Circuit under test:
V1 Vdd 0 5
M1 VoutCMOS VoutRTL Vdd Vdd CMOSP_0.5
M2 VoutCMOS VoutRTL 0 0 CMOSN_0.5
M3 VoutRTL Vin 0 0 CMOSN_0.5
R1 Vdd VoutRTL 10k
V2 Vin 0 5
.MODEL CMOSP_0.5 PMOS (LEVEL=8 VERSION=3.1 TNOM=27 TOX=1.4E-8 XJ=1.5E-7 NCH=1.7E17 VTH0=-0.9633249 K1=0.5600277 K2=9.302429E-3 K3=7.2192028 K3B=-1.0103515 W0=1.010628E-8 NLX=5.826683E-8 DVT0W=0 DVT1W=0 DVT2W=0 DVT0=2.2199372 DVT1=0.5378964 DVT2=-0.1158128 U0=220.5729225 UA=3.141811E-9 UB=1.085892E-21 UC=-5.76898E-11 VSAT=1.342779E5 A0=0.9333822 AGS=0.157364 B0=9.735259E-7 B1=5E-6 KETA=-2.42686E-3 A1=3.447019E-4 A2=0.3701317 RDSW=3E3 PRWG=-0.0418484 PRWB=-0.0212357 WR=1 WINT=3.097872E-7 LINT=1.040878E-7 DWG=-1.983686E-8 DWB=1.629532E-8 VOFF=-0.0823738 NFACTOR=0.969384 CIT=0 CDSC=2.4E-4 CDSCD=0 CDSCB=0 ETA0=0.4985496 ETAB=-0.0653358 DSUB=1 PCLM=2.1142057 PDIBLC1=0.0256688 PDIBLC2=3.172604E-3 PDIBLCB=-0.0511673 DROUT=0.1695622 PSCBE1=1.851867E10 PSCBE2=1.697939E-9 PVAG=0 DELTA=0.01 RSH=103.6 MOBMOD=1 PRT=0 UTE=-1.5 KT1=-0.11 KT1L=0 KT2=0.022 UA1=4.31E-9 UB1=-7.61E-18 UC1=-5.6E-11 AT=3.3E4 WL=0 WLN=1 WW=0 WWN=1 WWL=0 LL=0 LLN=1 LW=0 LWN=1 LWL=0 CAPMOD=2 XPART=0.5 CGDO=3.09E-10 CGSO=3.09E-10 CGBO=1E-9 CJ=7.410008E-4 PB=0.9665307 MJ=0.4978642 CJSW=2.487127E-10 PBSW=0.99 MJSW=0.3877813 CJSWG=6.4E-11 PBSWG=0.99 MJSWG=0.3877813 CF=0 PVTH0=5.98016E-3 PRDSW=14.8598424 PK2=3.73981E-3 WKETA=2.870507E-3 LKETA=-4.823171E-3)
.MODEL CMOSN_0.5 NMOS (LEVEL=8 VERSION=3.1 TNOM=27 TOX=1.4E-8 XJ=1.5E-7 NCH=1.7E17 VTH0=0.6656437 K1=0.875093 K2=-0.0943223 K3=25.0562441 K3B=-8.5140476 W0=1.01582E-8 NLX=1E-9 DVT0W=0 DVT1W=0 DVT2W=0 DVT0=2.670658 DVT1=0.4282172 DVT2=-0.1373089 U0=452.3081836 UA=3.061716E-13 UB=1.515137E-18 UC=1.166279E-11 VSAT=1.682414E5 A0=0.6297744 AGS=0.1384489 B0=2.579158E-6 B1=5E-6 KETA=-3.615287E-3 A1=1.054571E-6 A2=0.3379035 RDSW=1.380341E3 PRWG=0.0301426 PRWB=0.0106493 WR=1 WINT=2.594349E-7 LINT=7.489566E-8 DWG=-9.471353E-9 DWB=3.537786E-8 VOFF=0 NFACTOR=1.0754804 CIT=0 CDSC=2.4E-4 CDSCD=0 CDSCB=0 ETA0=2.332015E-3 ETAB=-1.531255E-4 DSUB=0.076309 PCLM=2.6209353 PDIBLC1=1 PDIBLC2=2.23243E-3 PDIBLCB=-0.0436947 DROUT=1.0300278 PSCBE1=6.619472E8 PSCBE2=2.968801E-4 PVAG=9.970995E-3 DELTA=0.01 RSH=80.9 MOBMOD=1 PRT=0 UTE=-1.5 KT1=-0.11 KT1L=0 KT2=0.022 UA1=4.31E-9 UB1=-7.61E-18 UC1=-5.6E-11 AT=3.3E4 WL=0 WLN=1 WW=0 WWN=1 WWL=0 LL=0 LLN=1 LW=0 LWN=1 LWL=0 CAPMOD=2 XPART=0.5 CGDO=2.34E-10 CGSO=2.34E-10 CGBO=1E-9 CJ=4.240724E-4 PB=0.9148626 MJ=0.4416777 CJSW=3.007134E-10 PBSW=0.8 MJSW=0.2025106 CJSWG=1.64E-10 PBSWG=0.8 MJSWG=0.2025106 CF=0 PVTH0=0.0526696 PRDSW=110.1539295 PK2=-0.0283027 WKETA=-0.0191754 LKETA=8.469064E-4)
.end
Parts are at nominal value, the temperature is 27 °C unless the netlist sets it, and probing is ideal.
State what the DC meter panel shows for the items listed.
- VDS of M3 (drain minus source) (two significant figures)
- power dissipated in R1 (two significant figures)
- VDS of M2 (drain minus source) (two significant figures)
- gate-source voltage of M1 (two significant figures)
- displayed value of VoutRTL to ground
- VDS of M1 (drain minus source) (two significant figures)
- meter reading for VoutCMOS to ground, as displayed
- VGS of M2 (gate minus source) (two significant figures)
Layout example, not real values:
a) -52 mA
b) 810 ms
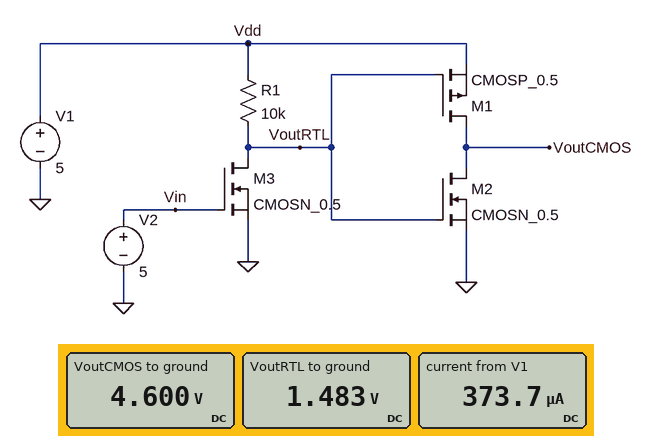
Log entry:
a) 1.5 V
b) 1.2 mW
c) 4.6 V
d) -3.5 V
e) 1.483 V
f) -400 mV
g) 4.600 V
h) 1.5 V
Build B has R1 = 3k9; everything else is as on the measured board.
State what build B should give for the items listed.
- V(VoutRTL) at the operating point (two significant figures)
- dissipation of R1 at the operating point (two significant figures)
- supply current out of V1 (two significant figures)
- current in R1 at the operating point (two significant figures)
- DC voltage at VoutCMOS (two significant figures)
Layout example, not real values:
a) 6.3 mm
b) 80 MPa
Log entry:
a) 3.0 V
b) 1.0 mW
c) 520 µA
d) 510 µA
e) 69 mV
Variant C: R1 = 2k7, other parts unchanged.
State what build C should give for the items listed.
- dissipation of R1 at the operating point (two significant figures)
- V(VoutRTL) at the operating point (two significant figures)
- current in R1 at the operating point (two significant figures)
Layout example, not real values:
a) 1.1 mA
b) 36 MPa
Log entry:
a) 730 µW
b) 3.6 V
c) 520 µA
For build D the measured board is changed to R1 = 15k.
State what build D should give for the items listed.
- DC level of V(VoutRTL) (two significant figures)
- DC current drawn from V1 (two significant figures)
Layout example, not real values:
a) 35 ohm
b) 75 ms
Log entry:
a) 1.0 V
b) 270 µA
